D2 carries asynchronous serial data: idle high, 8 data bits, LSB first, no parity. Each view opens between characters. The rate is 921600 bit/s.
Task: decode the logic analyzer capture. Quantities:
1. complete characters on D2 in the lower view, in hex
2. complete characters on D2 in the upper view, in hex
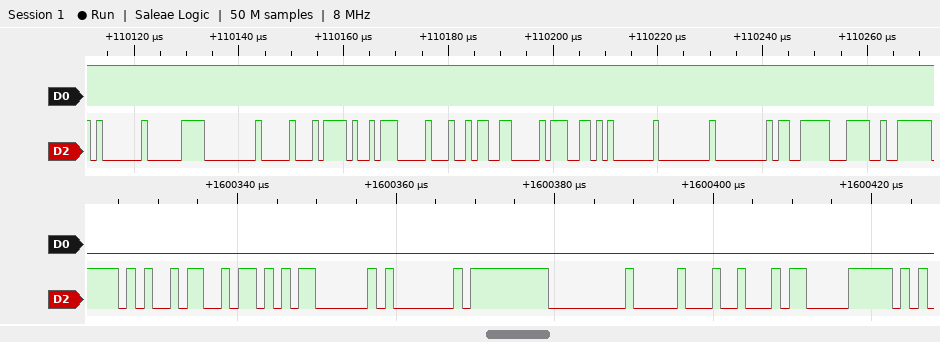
A5, 5A, 03, 01, FF, 00, 10, A2, F0
01, E0, 00, 10, 2F, 07, A4, 06, 67, 01, 00, 00, F3, 3C
